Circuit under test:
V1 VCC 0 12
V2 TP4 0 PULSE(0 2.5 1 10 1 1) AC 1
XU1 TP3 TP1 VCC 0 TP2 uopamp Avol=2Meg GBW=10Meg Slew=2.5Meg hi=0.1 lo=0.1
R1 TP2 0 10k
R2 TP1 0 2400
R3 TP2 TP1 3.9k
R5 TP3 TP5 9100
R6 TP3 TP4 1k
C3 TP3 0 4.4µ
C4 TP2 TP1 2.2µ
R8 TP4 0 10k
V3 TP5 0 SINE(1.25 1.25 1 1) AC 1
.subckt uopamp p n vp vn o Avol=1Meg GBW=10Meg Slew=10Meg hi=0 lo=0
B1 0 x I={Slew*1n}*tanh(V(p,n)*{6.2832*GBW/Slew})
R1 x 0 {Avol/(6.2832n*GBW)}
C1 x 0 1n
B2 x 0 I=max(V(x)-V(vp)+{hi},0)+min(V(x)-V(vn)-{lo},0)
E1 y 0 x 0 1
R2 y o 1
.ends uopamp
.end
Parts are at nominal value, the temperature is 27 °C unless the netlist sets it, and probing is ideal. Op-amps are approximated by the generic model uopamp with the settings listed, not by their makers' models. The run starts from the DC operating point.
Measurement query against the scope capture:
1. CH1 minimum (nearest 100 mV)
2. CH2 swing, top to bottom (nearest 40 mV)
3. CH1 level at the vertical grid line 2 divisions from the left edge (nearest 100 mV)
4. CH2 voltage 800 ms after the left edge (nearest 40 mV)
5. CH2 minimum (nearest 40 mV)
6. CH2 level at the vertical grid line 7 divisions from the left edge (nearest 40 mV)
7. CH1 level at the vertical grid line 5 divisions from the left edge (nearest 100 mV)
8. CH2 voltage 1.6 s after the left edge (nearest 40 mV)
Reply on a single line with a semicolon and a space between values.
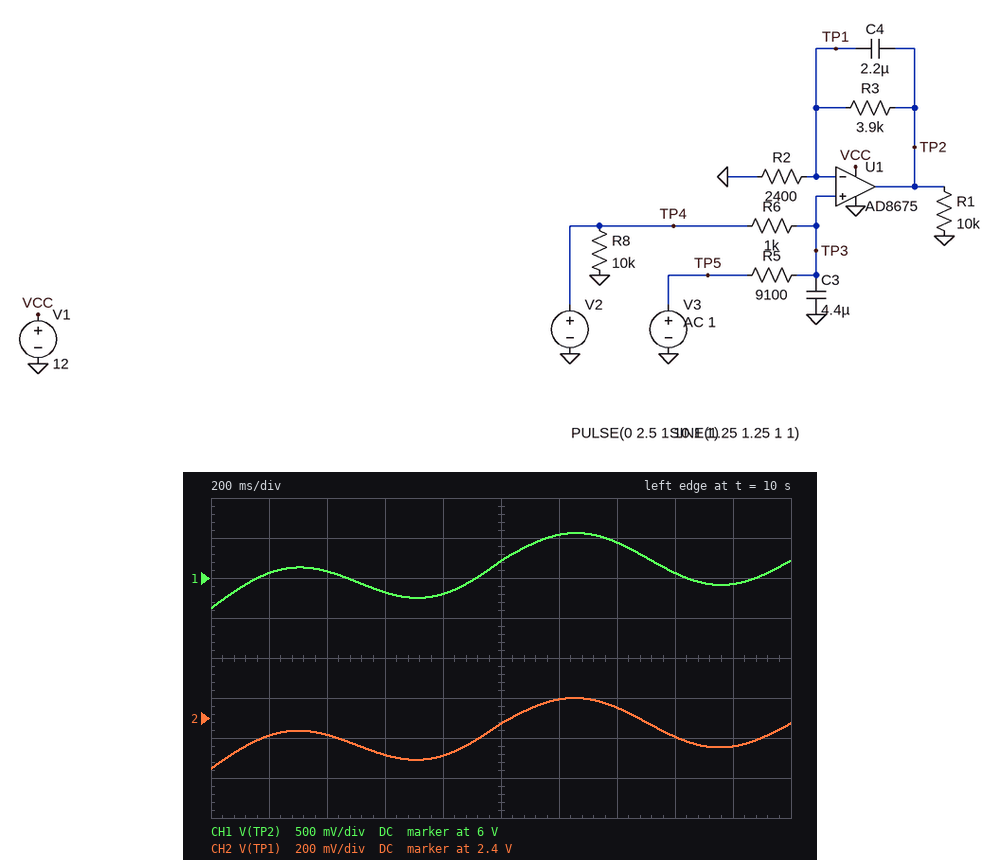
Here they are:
5.6 V; 360 mV; 6.1 V; 2.20 V; 2.16 V; 2.44 V; 6.2 V; 2.32 V
